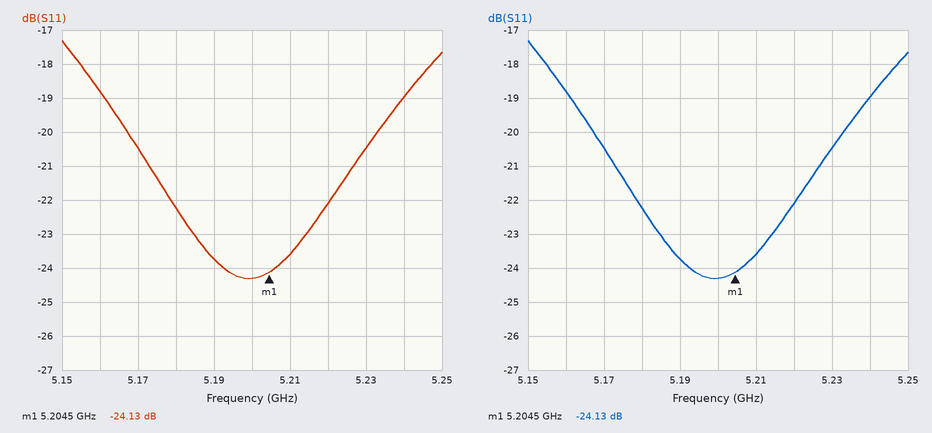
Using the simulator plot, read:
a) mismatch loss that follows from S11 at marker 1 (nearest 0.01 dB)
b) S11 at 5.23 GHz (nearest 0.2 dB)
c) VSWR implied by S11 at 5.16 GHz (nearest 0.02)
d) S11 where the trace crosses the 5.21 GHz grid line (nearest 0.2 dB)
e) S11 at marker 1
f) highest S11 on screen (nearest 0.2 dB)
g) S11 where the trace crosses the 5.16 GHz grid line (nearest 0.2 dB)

0.02 dB
-20.4 dB
1.26
-23.6 dB
-24.13 dB
-17.4 dB
-18.8 dB
